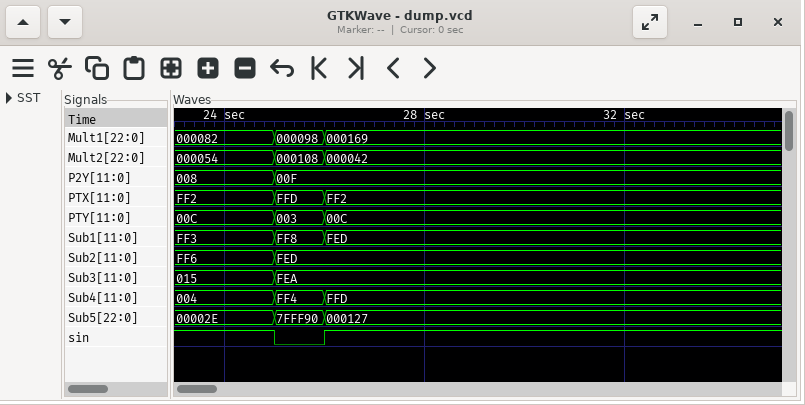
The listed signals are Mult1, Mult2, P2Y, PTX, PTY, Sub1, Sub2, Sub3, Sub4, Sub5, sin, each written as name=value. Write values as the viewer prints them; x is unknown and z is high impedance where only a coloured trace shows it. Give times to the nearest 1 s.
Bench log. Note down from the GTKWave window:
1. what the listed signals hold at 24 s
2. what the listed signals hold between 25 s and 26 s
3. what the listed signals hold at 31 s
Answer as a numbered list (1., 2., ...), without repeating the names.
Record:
1. Mult1=000082, Mult2=000054, P2Y=008, PTX=FF2, PTY=00C, Sub1=FF3, Sub2=FF6, Sub3=015, Sub4=004, Sub5=00002E, sin=1
2. Mult1=000098, Mult2=000108, P2Y=00F, PTX=FFD, PTY=003, Sub1=FF8, Sub2=FED, Sub3=FEA, Sub4=FF4, Sub5=7FFF90, sin=0
3. Mult1=000169, Mult2=000042, P2Y=00F, PTX=FF2, PTY=00C, Sub1=FED, Sub2=FED, Sub3=FEA, Sub4=FFD, Sub5=000127, sin=1
